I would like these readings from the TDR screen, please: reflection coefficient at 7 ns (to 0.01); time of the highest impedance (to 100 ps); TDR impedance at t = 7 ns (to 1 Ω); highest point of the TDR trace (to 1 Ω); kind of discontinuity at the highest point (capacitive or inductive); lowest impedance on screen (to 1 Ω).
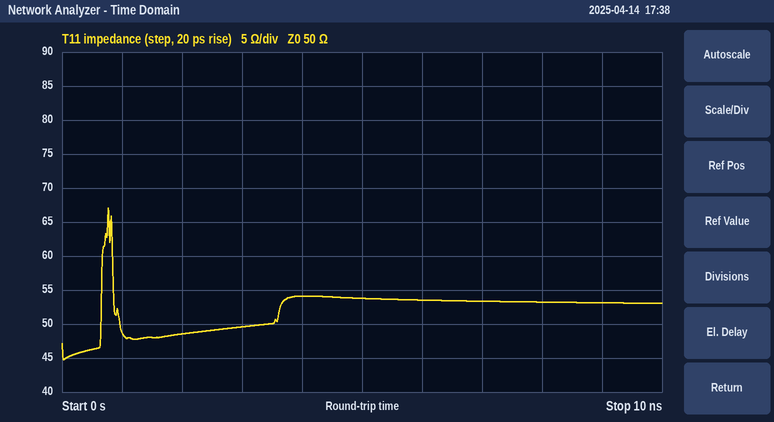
+0.03
800 ps
53 Ω
67 Ω
inductive
45 Ω
